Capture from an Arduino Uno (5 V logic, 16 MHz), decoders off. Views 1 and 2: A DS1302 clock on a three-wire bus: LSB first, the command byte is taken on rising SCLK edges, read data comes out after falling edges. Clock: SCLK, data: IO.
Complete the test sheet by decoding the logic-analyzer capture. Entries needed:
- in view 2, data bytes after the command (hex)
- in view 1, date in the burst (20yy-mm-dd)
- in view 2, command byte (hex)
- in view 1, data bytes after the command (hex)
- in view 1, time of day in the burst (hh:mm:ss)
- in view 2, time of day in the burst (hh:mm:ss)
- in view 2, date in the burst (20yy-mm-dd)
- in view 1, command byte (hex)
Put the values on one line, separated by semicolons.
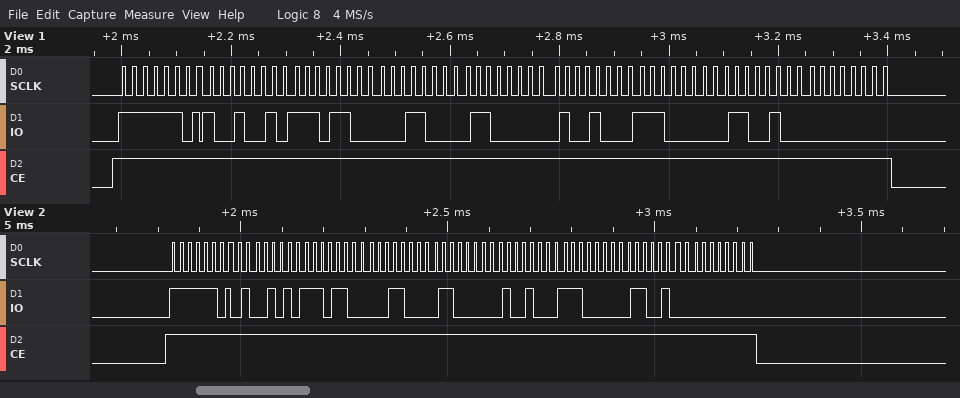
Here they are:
52 37 18 06 12 07 26 00; 2026-12-06; 0xBF; 49 37 18 06 12 07 26 00; 18:37:49; 18:37:52; 2026-12-06; 0xBF
